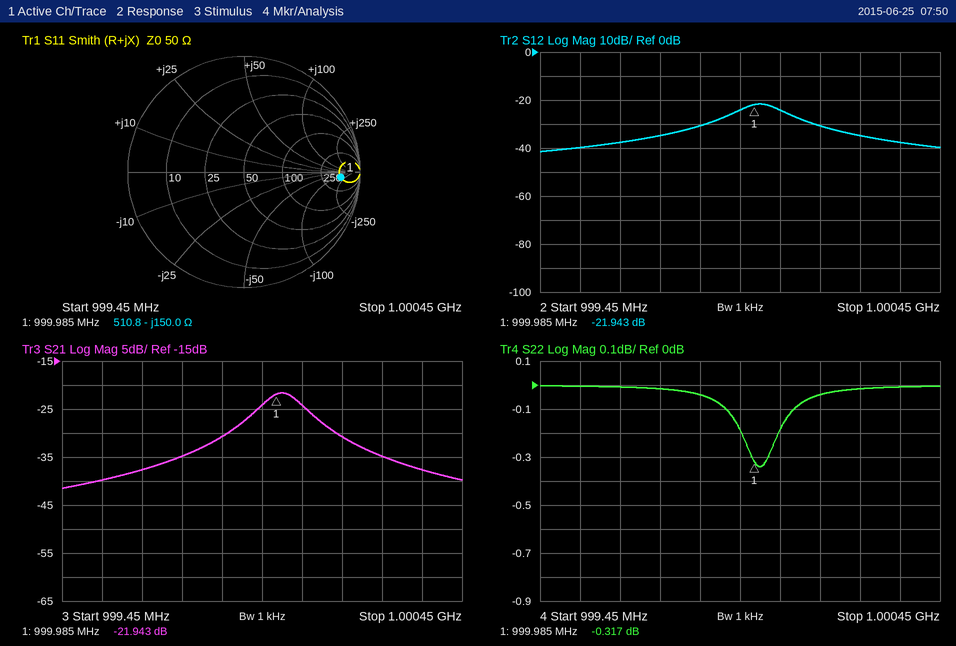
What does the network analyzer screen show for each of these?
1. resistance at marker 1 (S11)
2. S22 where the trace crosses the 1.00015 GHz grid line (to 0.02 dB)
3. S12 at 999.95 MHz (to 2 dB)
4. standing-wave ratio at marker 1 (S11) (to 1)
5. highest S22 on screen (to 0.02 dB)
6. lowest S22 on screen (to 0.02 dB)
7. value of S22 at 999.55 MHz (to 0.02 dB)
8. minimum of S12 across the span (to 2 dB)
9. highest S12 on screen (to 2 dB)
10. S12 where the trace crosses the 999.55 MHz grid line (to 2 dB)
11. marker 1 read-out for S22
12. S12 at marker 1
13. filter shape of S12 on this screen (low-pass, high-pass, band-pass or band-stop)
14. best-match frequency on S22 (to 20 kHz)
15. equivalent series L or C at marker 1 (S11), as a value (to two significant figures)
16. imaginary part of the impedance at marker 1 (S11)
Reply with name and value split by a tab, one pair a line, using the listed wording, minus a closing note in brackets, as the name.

resistance at marker 1	510.8 Ω
S22 where the trace crosses the 1.00015 GHz grid line	-0.04 dB
S12 at 999.95 MHz	-24 dB
standing-wave ratio at marker 1 (S11)	11
highest S22 on screen	0.00 dB
lowest S22 on screen	-0.34 dB
value of S22 at 999.55 MHz	0.00 dB
minimum of S12 across the span	-42 dB
highest S12 on screen	-22 dB
S12 where the trace crosses the 999.55 MHz grid line	-40 dB
marker 1 read-out for S22	-0.317 dB
S12 at marker 1	-21.943 dB
filter shape of S12 on this screen	band-pass
best-match frequency on S22	1.00000 GHz
equivalent series L or C at marker 1 (S11), as a value	1.1 pF
imaginary part of the impedance at marker 1	-150.0 Ω
